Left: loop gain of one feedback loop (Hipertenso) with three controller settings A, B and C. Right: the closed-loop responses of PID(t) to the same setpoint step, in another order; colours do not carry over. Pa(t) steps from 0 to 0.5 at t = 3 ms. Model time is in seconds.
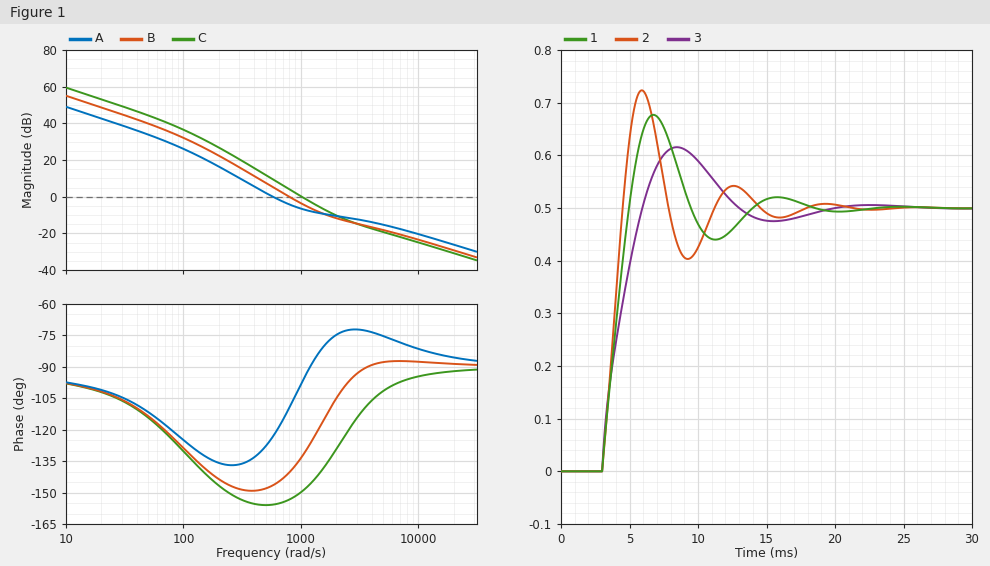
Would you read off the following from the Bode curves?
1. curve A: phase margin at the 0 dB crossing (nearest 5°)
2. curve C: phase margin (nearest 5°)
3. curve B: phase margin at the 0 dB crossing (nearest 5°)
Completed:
55°
30°
40°
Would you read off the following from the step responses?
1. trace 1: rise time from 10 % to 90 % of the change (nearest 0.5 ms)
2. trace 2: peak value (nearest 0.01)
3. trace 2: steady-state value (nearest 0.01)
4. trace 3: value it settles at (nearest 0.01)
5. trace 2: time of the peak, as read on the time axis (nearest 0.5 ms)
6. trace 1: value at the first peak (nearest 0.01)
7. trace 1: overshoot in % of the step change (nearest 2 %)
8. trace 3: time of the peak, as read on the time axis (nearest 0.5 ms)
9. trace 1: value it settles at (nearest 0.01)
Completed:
1.5 ms
0.72
0.50
0.50
6.0 ms
0.68
36 %
8.5 ms
0.50
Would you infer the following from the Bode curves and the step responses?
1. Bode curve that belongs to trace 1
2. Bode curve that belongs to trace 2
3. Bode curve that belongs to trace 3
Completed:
B
C
A
